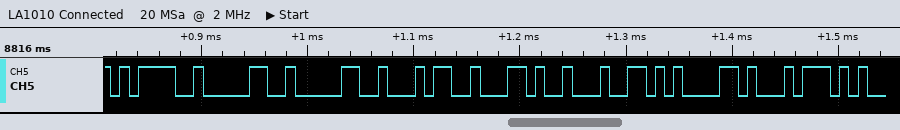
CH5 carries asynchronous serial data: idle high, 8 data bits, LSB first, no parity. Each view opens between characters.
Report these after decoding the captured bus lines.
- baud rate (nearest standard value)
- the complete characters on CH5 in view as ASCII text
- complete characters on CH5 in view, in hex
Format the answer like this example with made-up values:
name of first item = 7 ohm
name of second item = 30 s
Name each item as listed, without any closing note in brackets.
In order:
baud rate = 115200 baud
the complete characters on CH5 in view as ASCII text = "=004,dat"
complete characters on CH5 in view, in hex = 3D, 30, 30, 34, 2C, 64, 61, 74
